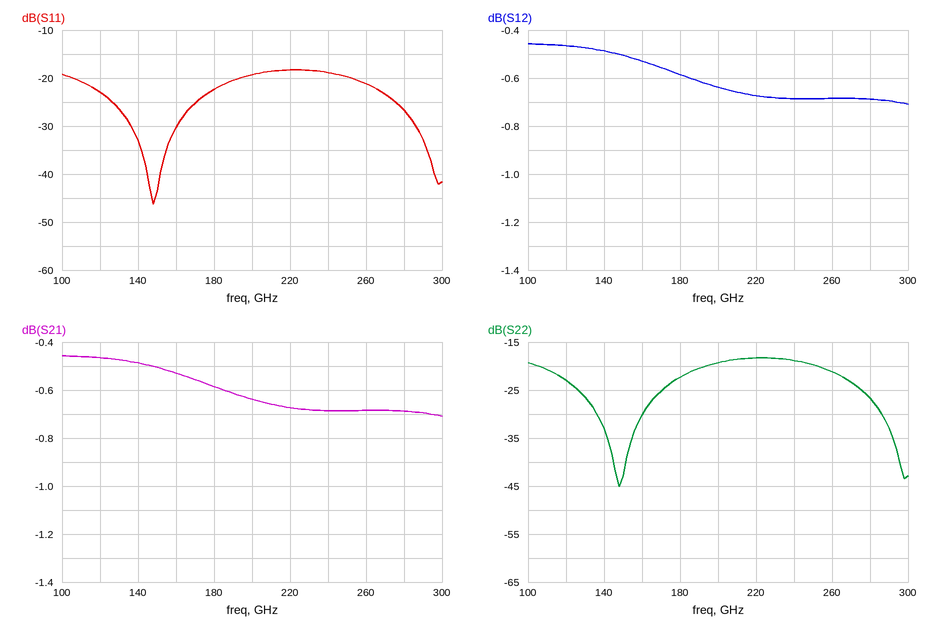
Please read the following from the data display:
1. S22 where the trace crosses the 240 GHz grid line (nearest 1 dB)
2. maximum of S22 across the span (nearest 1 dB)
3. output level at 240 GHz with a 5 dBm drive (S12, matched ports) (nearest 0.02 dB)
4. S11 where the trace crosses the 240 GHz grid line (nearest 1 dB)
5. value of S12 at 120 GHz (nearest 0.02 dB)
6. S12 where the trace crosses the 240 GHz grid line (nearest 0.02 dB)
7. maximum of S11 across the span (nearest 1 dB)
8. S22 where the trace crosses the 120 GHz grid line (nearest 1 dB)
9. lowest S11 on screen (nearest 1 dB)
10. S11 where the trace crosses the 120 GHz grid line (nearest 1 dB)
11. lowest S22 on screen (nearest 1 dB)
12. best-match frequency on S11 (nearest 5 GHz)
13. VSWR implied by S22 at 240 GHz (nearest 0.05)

-19 dB
-18 dB
4.32 dBm
-19 dB
-0.46 dB
-0.68 dB
-18 dB
-23 dB
-46 dB
-23 dB
-45 dB
150 GHz
1.25
